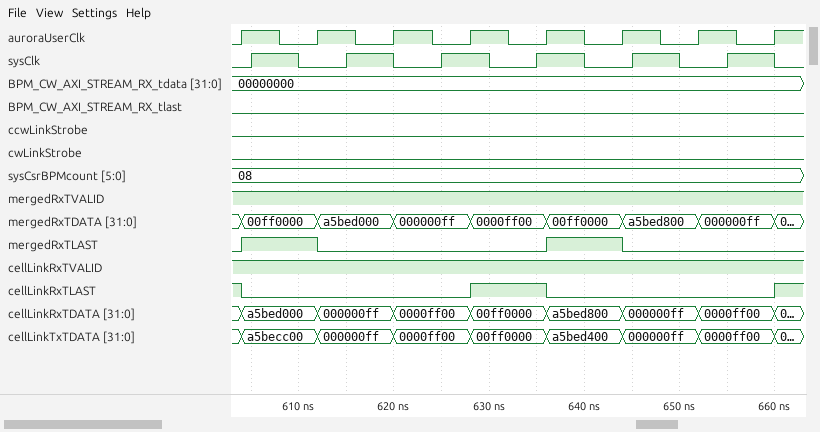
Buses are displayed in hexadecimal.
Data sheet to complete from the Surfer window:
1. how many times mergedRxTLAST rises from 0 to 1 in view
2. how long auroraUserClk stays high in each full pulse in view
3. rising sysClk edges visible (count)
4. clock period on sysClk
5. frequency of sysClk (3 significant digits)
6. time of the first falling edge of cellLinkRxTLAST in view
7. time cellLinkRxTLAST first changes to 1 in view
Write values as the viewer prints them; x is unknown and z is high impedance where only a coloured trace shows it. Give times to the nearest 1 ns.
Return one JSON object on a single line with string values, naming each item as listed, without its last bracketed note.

{"how many times mergedRxTLAST rises from 0 to 1 in view": "2", "how long auroraUserClk stays high in each full pulse in view": "4 ns, 4 ns, 4 ns, 4 ns, 4 ns, 4 ns, 4 ns", "rising sysClk edges visible": "6", "clock period on sysClk": "10 ns", "frequency of sysClk": "100 MHz", "time of the first falling edge of cellLinkRxTLAST in view": "604 ns", "time cellLinkRxTLAST first changes to 1 in view": "628 ns"}
